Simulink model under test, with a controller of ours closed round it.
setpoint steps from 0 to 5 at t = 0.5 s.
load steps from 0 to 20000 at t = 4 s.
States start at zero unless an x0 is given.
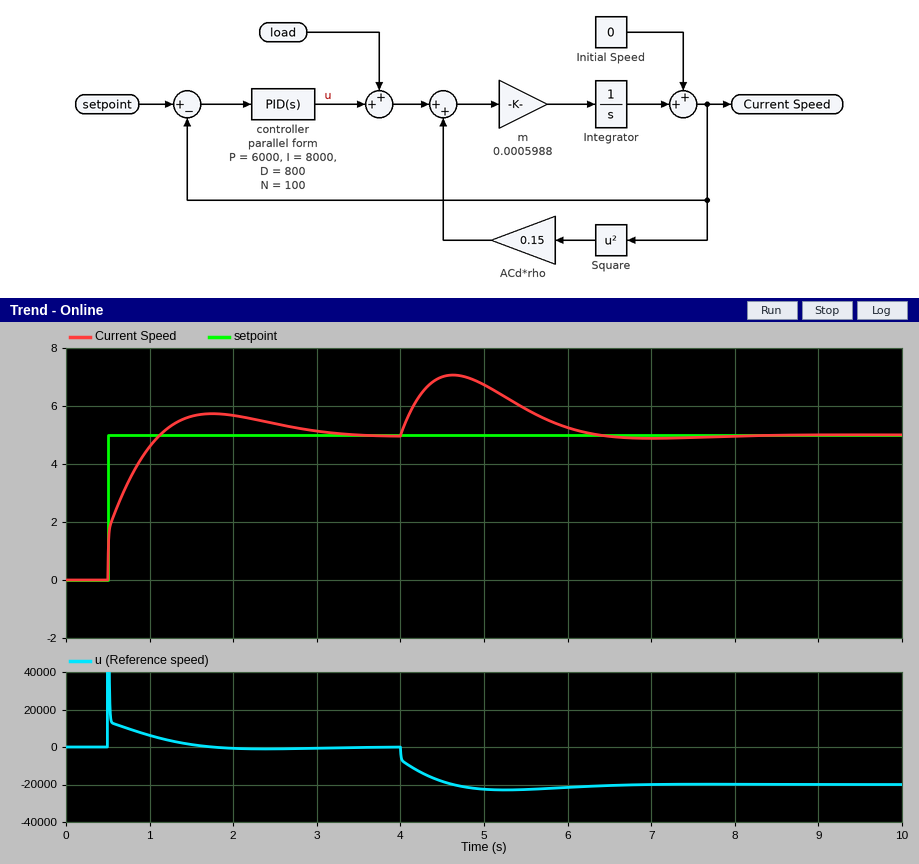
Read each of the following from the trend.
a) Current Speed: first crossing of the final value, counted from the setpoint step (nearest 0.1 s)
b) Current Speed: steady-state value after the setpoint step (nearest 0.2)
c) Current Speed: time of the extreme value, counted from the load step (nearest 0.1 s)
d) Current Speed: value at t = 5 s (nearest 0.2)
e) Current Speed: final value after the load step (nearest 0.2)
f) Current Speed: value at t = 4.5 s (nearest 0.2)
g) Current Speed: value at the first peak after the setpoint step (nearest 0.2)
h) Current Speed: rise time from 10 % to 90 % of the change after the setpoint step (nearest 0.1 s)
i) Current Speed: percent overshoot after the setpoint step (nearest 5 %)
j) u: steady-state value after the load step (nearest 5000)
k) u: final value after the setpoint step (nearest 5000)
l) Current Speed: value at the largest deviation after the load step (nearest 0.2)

0.6 s
5.0
0.6 s
6.8
5.0
7.0
5.8
0.5 s
15 %
-20000
0
7.0
